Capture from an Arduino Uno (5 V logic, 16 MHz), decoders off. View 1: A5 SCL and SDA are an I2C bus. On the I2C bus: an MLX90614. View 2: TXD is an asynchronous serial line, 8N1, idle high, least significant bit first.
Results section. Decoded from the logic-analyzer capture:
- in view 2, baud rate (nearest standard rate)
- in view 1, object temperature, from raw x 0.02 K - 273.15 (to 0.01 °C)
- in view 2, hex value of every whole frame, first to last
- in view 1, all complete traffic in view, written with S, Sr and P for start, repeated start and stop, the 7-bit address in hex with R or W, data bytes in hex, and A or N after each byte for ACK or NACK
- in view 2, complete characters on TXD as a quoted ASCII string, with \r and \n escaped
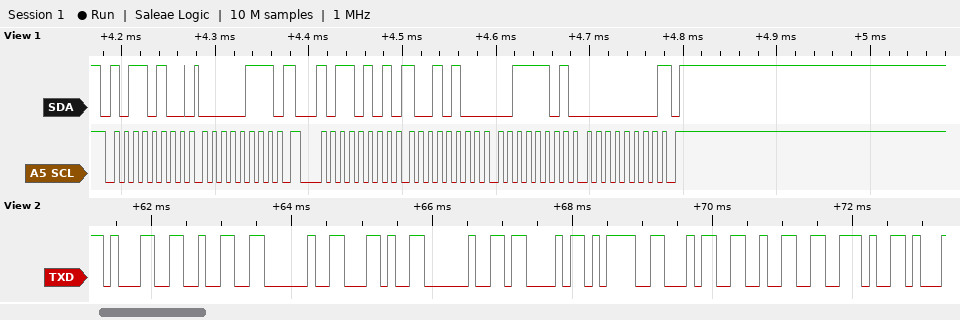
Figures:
9600 baud
42.13 °C
0x31 0x32 0x20 0x2C 0x20 0x43 0x3D 0x34 0x32 0x2E
S 5AW A 07 A Sr 5AR A 94 A 3D A 00 N P
"12 , C=42."
